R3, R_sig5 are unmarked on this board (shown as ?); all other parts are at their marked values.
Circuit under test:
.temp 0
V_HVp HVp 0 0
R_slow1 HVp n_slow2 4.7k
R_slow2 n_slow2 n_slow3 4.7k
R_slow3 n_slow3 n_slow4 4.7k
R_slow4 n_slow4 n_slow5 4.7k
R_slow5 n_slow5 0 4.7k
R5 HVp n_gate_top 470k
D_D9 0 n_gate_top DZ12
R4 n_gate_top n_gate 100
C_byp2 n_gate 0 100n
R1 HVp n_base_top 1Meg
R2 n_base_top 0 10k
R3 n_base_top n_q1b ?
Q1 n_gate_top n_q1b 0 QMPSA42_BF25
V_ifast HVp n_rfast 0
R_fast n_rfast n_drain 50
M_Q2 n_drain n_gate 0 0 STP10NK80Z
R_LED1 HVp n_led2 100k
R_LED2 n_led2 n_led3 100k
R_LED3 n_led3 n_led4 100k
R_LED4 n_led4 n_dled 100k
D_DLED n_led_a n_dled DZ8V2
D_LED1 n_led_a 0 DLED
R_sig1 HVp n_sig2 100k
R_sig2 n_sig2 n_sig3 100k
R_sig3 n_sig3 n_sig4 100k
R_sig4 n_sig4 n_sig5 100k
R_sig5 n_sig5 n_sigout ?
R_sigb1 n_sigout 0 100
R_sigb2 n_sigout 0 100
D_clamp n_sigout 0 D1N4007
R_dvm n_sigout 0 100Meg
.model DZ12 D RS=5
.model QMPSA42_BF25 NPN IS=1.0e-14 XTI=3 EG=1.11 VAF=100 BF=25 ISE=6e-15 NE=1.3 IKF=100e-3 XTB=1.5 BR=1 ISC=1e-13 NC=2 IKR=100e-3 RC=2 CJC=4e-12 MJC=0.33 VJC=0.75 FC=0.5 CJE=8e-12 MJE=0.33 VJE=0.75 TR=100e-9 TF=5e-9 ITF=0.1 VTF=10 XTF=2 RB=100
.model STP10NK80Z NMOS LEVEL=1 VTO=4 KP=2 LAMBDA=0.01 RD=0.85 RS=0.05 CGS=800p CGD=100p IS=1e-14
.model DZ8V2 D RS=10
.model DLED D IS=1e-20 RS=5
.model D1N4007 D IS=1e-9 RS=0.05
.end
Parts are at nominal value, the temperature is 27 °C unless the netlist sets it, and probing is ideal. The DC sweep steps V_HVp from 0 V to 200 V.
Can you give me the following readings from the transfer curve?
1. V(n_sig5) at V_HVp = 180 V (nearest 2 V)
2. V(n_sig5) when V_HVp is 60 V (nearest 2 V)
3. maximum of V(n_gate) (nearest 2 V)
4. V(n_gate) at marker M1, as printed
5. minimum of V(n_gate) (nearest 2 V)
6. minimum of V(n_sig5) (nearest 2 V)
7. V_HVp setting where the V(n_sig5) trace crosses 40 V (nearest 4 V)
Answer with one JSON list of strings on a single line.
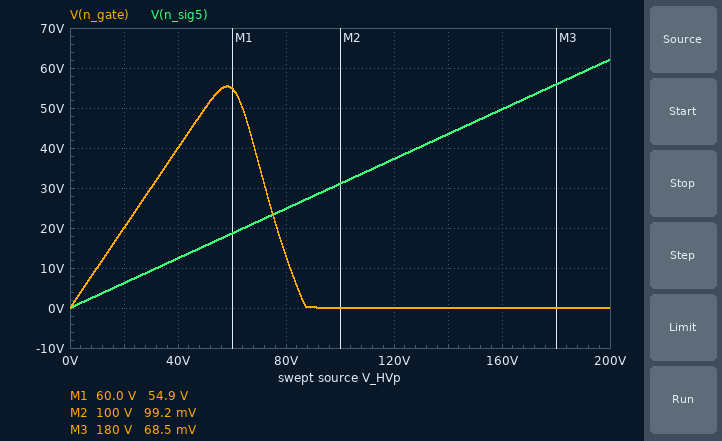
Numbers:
["56 V", "18 V", "56 V", "54.9 V", "0 V", "0 V", "128 V"]
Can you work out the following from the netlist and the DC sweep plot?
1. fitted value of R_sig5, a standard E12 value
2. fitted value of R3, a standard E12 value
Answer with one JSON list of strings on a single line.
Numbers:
["180 kΩ", "12 kΩ"]
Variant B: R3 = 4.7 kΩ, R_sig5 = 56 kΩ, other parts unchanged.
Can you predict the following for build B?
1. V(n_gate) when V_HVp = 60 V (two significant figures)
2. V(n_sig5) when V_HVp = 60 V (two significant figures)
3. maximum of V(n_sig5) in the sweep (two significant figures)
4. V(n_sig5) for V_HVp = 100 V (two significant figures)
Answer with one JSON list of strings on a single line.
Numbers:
["54 V", "7.4 V", "25 V", "12 V"]
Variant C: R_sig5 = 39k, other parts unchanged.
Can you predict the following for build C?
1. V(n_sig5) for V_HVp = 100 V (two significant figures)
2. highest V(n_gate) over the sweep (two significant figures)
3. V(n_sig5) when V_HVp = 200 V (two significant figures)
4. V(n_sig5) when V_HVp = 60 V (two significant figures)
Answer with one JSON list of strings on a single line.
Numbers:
["8.9 V", "55 V", "18 V", "5.3 V"]
